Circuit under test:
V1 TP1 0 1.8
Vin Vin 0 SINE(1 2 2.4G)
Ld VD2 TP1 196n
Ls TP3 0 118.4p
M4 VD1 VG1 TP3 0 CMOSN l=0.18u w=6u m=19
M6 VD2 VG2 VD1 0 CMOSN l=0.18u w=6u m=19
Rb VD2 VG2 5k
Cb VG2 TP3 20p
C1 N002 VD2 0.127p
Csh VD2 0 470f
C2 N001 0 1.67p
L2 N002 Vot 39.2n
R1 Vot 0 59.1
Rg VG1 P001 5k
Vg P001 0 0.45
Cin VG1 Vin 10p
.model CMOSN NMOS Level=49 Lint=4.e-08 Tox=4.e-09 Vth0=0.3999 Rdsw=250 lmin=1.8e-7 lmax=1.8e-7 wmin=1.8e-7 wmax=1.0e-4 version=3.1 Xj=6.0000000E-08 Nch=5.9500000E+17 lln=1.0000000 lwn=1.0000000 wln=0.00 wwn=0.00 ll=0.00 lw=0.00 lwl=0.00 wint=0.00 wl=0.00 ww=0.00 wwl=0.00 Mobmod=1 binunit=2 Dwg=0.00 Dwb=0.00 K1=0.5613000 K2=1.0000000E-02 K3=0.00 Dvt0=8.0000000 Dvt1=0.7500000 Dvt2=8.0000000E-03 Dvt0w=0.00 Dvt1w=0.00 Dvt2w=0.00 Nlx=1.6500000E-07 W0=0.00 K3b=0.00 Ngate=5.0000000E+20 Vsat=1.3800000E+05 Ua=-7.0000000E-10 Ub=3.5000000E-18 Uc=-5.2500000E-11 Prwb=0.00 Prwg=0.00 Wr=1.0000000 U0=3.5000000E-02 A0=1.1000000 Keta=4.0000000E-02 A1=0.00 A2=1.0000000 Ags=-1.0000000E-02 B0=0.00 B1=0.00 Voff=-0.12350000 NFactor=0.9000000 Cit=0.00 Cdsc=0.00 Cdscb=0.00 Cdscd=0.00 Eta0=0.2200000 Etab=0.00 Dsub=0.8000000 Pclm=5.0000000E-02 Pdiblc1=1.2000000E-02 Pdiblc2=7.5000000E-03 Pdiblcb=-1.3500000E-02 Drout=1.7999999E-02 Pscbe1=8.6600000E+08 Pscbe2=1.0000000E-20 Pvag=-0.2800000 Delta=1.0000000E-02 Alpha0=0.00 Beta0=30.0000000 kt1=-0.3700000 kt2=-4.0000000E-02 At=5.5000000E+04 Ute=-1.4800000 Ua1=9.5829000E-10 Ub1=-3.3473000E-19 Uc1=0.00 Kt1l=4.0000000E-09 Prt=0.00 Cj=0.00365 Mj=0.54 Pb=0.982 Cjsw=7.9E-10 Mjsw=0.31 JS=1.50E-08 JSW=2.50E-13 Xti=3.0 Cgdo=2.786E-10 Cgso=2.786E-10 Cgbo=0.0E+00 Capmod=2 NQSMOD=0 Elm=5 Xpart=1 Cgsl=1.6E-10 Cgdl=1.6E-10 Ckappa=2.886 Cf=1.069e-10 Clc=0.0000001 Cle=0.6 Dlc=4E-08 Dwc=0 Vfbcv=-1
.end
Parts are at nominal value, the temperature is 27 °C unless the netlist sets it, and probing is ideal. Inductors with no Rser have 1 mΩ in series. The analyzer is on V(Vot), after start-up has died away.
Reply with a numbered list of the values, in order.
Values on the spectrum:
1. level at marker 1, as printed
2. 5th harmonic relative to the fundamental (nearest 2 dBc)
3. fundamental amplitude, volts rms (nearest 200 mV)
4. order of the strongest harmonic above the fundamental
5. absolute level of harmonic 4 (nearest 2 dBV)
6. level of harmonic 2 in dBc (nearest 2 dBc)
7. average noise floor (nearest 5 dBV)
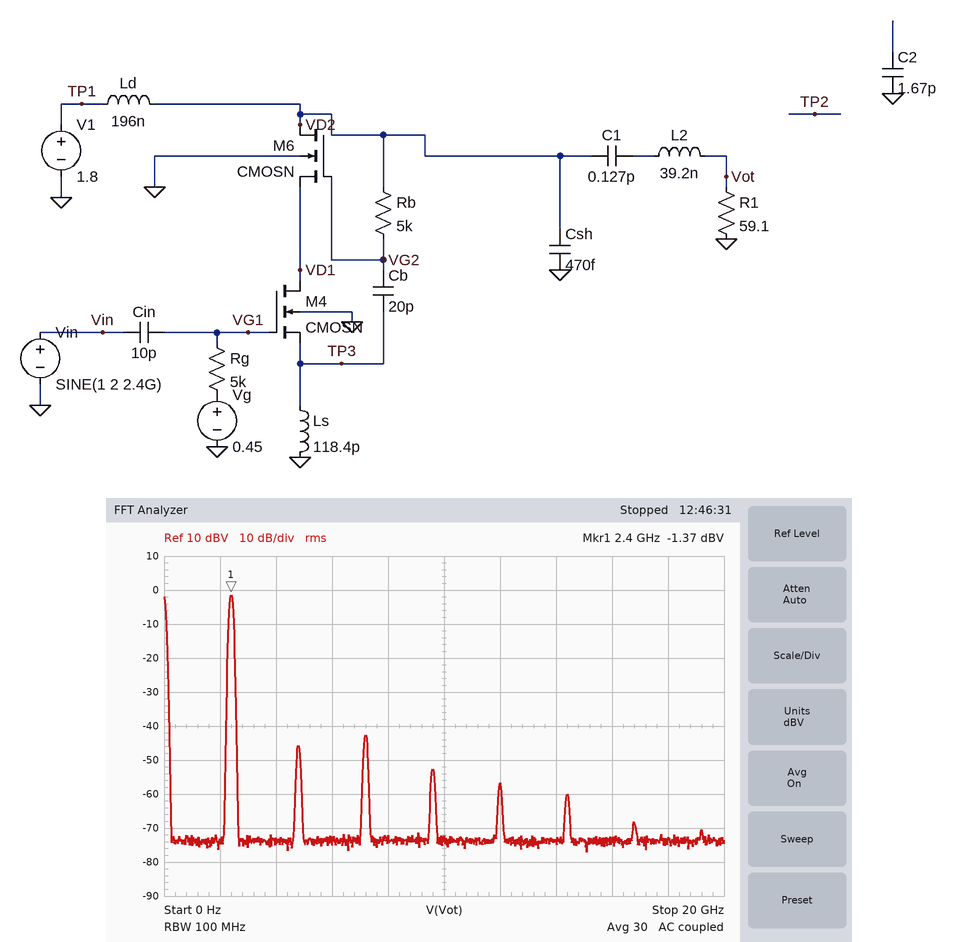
1. -1.37 dBV
2. -56 dBc
3. 800 mV
4. 3
5. -52 dBV
6. -44 dBc
7. -75 dBV
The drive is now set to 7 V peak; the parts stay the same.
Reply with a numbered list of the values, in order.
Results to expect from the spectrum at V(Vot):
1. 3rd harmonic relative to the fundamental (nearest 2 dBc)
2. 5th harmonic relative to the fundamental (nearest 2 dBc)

1. -40 dBc
2. -52 dBc
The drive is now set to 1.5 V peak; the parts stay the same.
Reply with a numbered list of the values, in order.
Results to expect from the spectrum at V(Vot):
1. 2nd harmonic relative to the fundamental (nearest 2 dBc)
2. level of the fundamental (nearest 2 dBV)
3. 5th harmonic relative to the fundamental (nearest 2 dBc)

1. -48 dBc
2. -2 dBV
3. -58 dBc
